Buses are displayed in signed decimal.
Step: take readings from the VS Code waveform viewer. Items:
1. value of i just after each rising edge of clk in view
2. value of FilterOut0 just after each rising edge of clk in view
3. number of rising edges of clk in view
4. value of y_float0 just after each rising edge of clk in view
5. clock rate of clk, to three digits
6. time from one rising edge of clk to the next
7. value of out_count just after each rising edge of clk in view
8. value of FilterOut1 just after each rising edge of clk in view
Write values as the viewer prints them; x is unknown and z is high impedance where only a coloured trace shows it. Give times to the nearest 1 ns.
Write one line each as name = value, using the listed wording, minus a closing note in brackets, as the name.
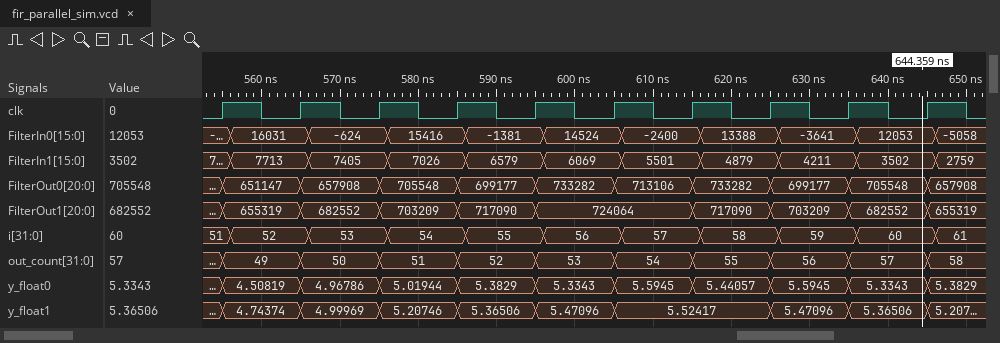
value of i just after each rising edge of clk in view = 51, 52, 53, 54, 55, 56, 57, 58, 59, 60
value of FilterOut0 just after each rising edge of clk in view = 651147, 657908, 705548, 699177, 733282, 713106, 733282, 699177, 705548, 657908
number of rising edges of clk in view = 10
value of y_float0 just after each rising edge of clk in view = 4.50819, 4.96786, 5.01944, 5.3829, 5.3343, 5.5945, 5.44057, 5.5945, 5.3343, 5.3829
clock rate of clk, to three digits = 100 MHz
time from one rising edge of clk to the next = 10 ns
value of out_count just after each rising edge of clk in view = 49, 50, 51, 52, 53, 54, 55, 56, 57, 58
value of FilterOut1 just after each rising edge of clk in view = 655319, 682552, 703209, 717090, 724064, 724064, 717090, 703209, 682552, 655319
